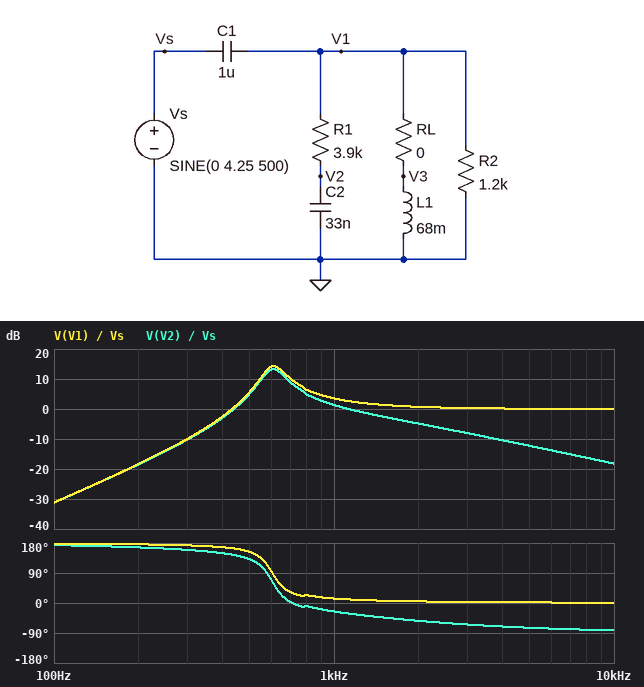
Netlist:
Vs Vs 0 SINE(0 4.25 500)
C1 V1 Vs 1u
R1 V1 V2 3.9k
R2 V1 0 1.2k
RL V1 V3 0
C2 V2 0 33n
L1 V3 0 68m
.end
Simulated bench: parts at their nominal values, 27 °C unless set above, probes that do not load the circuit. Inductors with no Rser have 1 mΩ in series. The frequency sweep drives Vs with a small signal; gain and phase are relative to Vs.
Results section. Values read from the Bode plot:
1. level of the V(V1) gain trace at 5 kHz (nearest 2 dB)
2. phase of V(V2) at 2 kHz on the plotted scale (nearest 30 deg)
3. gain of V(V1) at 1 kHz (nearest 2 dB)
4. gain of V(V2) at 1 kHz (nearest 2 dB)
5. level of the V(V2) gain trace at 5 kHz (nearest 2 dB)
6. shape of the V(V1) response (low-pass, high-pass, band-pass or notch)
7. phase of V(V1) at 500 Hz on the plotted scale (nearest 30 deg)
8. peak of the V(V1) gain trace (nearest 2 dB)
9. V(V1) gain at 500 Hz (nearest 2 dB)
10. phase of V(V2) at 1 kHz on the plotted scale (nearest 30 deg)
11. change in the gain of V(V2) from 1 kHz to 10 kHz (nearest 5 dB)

0 dB
-60 deg
4 dB
2 dB
-12 dB
high-pass
150 deg
14 dB
6 dB
-30 deg
-20 dB
